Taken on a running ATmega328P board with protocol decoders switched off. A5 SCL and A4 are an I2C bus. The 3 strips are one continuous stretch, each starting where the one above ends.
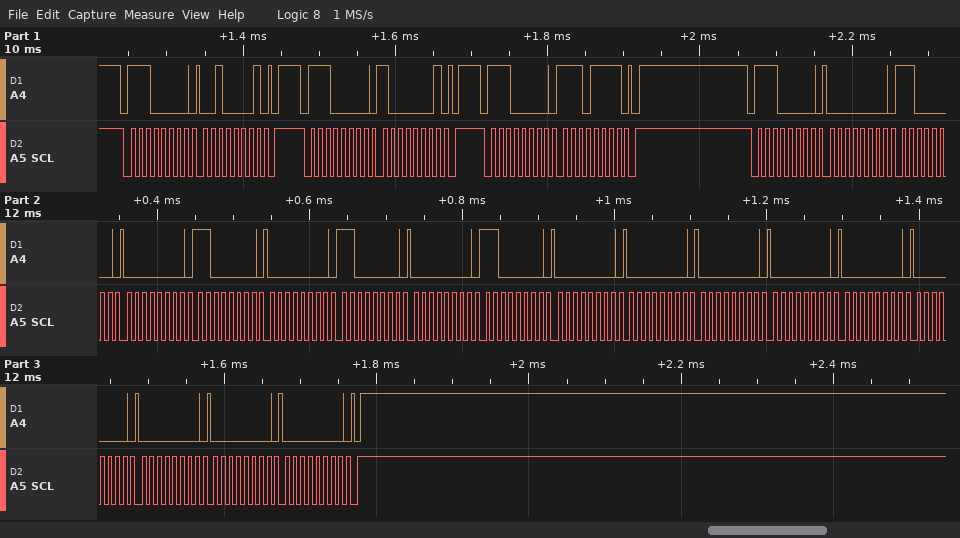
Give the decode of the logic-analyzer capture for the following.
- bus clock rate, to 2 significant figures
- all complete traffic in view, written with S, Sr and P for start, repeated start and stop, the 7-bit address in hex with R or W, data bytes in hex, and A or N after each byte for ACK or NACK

100 kHz
S 70W A 21 A P S 70W A 81 A P S 70W A EF A P S 70W A 00 A C0 A 00 A C0 A 00 A C0 A 00 A C0 A 00 A 00 A 00 A 00 A 00 A 00 A 00 A 00 A 00 A P
